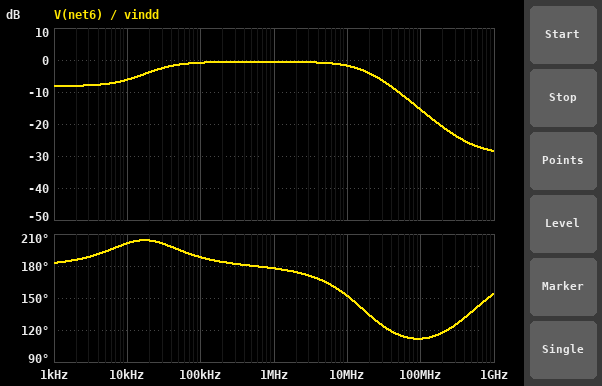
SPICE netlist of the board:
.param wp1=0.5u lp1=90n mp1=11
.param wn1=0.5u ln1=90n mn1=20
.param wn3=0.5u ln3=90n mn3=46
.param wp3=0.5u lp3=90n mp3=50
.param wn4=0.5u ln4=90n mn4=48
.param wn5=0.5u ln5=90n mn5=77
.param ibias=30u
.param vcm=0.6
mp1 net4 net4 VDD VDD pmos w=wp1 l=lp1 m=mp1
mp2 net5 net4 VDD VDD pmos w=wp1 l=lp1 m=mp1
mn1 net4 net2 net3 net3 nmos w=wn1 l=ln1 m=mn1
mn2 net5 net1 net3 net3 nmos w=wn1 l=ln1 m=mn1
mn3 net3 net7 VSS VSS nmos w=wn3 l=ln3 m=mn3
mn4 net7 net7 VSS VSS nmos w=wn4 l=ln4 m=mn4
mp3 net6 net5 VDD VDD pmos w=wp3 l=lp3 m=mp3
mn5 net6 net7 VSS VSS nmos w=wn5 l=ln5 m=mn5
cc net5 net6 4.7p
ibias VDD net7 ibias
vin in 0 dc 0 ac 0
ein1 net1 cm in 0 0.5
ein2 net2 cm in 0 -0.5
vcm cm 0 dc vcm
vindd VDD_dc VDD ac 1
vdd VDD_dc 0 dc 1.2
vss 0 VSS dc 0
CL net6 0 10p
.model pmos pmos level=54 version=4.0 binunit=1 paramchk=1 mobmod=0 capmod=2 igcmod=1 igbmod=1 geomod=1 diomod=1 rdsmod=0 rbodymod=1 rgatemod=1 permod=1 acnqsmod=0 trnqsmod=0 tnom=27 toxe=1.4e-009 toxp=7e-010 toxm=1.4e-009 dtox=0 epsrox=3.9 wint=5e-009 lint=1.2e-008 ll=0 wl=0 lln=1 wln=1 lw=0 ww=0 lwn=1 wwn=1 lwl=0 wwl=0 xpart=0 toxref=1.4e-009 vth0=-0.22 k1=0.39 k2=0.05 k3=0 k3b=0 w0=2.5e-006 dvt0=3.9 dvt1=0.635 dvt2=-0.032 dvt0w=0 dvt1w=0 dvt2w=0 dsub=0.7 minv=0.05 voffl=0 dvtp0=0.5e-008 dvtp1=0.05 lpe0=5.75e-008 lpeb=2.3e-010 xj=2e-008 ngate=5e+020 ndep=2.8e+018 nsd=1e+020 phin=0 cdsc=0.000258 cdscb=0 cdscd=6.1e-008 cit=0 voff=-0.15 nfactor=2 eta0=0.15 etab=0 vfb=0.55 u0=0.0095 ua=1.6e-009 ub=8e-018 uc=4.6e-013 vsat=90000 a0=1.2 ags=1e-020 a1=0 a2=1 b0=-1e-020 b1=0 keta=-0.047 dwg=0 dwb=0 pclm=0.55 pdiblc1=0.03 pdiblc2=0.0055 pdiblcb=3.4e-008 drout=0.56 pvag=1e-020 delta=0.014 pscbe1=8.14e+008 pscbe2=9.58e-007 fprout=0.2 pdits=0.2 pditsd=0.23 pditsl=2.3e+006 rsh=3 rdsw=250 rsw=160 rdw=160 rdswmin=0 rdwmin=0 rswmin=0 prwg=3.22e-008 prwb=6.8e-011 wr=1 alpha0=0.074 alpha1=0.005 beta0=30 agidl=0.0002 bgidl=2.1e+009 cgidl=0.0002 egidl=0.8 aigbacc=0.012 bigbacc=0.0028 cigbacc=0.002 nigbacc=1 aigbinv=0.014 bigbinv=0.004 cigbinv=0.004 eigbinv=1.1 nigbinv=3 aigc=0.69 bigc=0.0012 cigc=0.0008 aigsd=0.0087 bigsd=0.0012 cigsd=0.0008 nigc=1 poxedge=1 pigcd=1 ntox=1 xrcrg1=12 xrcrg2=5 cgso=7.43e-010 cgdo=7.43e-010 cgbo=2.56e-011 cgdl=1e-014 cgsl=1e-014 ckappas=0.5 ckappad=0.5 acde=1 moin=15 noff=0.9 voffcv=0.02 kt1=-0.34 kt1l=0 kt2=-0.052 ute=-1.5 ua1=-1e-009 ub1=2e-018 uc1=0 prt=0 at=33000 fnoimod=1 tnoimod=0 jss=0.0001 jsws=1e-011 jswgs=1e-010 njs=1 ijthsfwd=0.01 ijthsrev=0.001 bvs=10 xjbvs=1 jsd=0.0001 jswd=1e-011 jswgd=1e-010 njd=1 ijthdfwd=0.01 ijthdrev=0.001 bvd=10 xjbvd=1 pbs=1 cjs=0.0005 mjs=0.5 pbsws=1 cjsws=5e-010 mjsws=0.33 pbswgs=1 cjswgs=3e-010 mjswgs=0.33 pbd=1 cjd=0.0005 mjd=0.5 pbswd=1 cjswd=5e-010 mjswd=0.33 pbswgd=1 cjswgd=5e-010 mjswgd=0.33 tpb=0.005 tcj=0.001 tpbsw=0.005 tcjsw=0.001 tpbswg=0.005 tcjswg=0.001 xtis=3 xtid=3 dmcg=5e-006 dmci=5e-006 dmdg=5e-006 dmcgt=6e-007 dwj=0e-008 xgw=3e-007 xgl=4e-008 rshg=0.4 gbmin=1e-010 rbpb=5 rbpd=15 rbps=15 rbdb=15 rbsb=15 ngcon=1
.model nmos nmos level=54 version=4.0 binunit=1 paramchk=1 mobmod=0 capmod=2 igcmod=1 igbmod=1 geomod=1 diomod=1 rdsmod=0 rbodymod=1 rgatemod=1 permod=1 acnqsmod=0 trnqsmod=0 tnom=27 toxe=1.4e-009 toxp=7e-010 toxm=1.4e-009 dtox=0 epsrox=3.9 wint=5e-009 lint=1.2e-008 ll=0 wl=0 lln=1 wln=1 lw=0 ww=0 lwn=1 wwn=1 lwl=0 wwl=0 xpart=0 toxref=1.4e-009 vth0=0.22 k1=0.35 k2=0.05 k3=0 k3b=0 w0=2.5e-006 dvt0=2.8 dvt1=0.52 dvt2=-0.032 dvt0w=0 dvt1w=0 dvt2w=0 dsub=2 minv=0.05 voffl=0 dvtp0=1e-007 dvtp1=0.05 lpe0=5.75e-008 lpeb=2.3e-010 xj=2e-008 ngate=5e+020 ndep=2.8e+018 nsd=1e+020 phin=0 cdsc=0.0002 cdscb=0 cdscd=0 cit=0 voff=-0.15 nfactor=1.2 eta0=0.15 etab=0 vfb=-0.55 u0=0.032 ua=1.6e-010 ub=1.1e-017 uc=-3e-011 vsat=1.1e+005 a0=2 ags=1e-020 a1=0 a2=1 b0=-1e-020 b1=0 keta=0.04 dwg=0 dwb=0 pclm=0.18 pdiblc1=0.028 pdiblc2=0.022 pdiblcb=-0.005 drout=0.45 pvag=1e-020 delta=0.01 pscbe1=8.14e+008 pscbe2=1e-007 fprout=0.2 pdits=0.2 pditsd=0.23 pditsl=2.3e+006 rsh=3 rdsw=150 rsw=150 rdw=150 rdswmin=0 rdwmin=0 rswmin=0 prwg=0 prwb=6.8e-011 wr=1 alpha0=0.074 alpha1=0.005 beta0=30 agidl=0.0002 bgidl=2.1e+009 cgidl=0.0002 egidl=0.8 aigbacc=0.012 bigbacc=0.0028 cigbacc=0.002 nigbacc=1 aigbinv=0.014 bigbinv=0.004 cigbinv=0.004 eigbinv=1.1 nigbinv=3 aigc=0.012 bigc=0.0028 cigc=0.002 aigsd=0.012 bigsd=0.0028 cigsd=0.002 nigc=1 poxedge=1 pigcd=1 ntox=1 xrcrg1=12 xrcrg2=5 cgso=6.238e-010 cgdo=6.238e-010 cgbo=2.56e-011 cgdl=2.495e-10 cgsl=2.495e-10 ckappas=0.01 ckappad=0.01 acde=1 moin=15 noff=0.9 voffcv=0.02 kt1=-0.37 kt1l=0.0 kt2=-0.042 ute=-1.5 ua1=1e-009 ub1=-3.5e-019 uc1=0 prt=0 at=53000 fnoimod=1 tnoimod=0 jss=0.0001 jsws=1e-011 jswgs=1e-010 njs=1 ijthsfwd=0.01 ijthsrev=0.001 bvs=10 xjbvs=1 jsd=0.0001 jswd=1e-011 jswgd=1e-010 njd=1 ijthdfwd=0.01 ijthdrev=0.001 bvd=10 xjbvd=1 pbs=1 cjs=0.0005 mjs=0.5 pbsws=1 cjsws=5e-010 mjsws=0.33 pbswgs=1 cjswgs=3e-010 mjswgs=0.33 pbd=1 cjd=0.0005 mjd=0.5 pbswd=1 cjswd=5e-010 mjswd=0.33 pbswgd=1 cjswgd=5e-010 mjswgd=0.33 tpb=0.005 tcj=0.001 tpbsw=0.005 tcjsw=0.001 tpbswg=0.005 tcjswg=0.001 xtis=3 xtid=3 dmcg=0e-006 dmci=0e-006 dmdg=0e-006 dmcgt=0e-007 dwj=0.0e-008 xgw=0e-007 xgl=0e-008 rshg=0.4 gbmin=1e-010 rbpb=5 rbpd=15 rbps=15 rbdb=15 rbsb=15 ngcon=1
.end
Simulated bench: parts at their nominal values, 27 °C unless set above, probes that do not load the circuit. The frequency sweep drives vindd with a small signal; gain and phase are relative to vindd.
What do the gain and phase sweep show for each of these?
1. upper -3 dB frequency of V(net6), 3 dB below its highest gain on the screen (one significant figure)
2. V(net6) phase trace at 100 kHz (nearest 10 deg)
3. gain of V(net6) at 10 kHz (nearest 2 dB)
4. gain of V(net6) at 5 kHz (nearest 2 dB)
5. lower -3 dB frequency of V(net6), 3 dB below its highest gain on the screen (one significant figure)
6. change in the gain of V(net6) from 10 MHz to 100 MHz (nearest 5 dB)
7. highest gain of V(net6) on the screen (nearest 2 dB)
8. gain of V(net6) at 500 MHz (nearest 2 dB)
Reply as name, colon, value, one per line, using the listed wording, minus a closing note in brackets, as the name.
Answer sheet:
upper -3 dB frequency of V(net6), 3 dB below its highest gain on the screen: 20 MHz
V(net6) phase trace at 100 kHz: 190 deg
gain of V(net6) at 10 kHz: -6 dB
gain of V(net6) at 5 kHz: -8 dB
lower -3 dB frequency of V(net6), 3 dB below its highest gain on the screen: 20 kHz
change in the gain of V(net6) from 10 MHz to 100 MHz: -15 dB
highest gain of V(net6) on the screen: 0 dB
gain of V(net6) at 500 MHz: -26 dB
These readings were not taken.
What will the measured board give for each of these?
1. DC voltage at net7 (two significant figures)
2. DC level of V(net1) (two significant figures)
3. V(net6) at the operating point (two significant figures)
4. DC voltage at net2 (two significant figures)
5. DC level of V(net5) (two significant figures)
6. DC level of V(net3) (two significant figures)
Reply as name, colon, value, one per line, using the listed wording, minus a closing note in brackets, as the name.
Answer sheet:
DC voltage at net7: 300 mV
DC level of V(net1): 600 mV
V(net6) at the operating point: 760 mV
DC voltage at net2: 600 mV
DC level of V(net5): 830 mV
DC level of V(net3): 300 mV
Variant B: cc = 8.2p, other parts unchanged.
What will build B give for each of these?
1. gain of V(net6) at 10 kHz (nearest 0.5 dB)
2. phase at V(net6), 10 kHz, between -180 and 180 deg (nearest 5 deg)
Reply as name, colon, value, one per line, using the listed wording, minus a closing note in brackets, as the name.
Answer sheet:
gain of V(net6) at 10 kHz: -4.5 dB
phase at V(net6), 10 kHz, between -180 and 180 deg: -155 deg
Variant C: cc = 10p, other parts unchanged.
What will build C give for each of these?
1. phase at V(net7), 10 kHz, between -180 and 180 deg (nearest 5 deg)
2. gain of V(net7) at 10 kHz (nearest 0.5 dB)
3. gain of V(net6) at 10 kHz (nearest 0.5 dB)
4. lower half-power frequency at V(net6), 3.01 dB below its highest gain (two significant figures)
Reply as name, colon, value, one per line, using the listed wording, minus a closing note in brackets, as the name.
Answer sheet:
phase at V(net7), 10 kHz, between -180 and 180 deg: -155 deg
gain of V(net7) at 10 kHz: -50.5 dB
gain of V(net6) at 10 kHz: -3.5 dB
lower half-power frequency at V(net6), 3.01 dB below its highest gain: 10 kHz
